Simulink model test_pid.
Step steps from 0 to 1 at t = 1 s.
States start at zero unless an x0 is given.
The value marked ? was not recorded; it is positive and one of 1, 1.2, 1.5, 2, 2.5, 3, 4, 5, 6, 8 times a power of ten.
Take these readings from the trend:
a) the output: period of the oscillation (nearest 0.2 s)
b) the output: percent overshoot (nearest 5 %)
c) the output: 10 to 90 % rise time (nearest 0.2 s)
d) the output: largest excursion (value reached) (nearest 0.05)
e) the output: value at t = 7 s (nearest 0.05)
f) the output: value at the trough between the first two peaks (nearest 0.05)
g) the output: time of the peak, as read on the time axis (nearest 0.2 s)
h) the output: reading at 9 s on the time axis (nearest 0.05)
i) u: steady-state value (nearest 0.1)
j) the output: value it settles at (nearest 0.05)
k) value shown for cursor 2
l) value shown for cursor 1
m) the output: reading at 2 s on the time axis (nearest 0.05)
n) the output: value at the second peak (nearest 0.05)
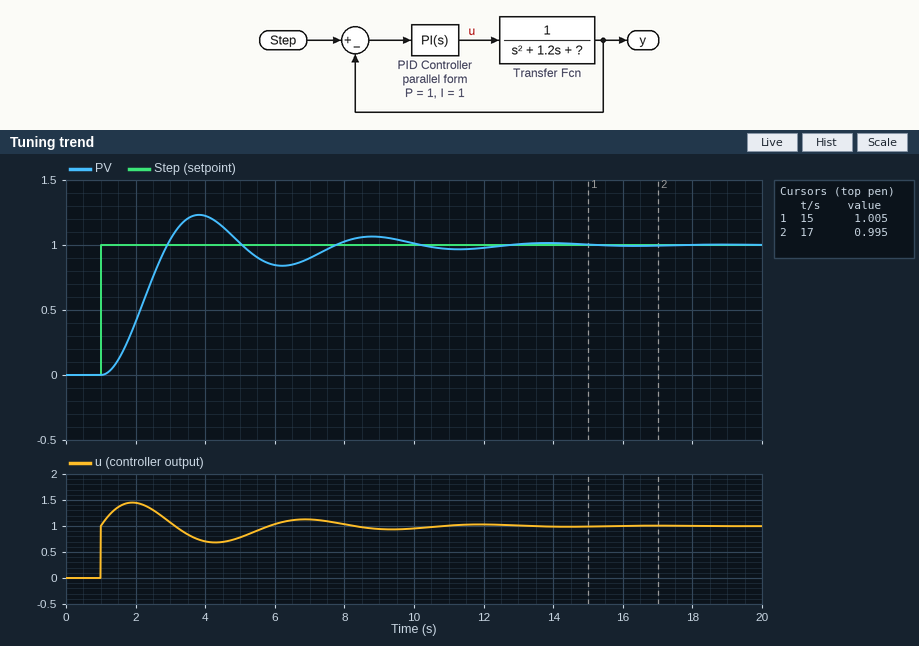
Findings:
5.0 s
25 %
1.2 s
1.25
0.90
0.85
3.8 s
1.05
1.0
1.00
0.995
1.005
0.40
1.05
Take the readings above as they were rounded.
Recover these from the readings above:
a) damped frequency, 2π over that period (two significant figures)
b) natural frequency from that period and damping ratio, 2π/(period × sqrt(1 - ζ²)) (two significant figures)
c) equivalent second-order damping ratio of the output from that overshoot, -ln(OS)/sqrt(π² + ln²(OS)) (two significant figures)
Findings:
1.3 rad/s
1.4 rad/s
0.40
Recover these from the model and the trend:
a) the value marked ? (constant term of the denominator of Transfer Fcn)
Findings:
1
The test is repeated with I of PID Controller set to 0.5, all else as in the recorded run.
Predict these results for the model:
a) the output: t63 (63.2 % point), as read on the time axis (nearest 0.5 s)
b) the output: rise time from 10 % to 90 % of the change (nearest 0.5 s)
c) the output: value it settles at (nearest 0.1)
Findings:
2.5 s
2.0 s
1.0
